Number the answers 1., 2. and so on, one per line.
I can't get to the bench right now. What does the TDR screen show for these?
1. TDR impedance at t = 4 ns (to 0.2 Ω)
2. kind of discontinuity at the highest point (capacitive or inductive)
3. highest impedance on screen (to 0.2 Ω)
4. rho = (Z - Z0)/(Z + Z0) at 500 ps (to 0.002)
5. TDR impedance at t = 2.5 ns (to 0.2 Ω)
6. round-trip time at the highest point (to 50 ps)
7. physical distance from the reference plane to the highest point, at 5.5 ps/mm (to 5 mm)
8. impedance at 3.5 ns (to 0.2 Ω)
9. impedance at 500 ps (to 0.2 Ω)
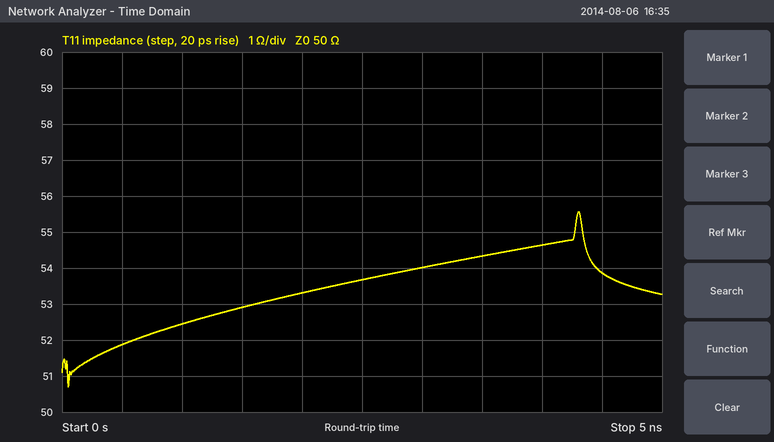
1. 54.6 Ω
2. inductive
3. 55.6 Ω
4. +0.018
5. 53.6 Ω
6. 4.30 ns
7. 390 mm
8. 54.4 Ω
9. 51.8 Ω
